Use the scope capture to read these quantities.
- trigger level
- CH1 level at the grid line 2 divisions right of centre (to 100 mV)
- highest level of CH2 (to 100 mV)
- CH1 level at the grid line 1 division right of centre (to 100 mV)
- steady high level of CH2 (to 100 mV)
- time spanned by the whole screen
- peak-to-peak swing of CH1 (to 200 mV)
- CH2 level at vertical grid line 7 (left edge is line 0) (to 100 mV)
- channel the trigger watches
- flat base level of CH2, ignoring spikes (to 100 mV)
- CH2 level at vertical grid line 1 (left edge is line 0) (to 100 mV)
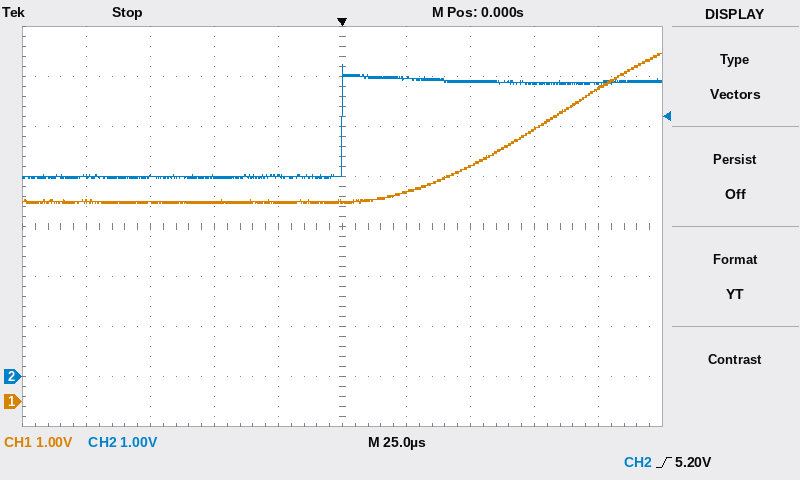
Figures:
5.20 V
4.7 V
6.2 V
4.2 V
5.9 V
250 µs
3.0 V
5.9 V
CH2
4.0 V
4.0 V
